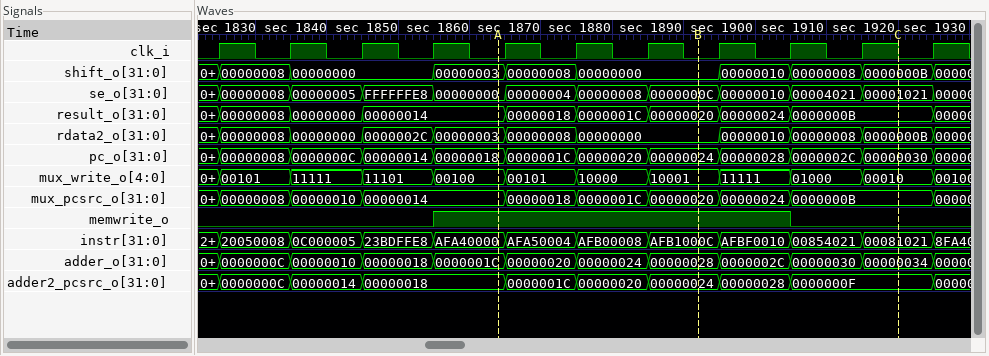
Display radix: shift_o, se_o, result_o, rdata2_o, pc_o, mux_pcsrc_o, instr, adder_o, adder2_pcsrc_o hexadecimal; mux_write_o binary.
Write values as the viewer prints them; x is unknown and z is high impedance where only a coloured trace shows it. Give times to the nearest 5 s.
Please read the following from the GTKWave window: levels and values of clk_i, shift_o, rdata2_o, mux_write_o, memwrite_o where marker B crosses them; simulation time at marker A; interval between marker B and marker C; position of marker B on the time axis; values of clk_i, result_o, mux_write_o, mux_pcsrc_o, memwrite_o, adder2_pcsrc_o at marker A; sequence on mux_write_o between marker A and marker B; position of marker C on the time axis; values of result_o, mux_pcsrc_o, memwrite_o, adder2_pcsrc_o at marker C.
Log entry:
clk_i=0, shift_o=00000000, rdata2_o=00000000, mux_write_o=10001, memwrite_o=1
1865 s
30 s
1890 s
clk_i=0, result_o=00000014, mux_write_o=00100, mux_pcsrc_o=00000014, memwrite_o=1, adder2_pcsrc_o=00000018
00100, 00101, 10000, 10001
1920 s
result_o=0000000B, mux_pcsrc_o=0000000B, memwrite_o=0, adder2_pcsrc_o=0000000F
